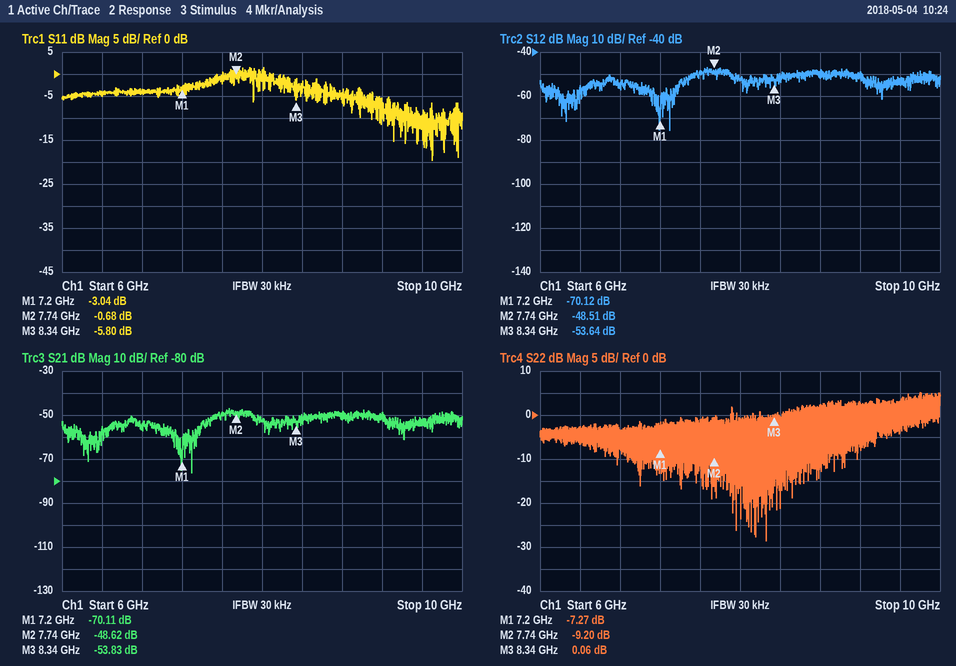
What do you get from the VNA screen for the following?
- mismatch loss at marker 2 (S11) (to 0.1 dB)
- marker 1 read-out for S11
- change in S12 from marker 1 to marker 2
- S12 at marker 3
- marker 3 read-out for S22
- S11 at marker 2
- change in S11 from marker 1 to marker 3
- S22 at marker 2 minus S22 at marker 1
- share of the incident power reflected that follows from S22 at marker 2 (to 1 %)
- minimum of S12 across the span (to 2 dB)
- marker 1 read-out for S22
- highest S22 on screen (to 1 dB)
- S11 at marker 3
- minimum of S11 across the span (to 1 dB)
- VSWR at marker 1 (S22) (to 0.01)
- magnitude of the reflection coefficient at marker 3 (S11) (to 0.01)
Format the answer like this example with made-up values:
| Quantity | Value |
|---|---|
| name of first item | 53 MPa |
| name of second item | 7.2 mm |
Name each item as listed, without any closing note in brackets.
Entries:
| Quantity | Value |
|---|---|
| mismatch loss at marker 2 (S11) | 8.4 dB |
| marker 1 read-out for S11 | -3.04 dB |
| change in S12 from marker 1 to marker 2 | 21.61 dB |
| S12 at marker 3 | -53.64 dB |
| marker 3 read-out for S22 | 0.06 dB |
| S11 at marker 2 | -0.68 dB |
| change in S11 from marker 1 to marker 3 | -2.76 dB |
| S22 at marker 2 minus S22 at marker 1 | -1.93 dB |
| share of the incident power reflected that follows from S22 at marker 2 | 12 % |
| minimum of S12 across the span | -76 dB |
| marker 1 read-out for S22 | -7.27 dB |
| highest S22 on screen | 5 dB |
| S11 at marker 3 | -5.80 dB |
| minimum of S11 across the span | -20 dB |
| VSWR at marker 1 (S22) | 2.53 |
| magnitude of the reflection coefficient at marker 3 (S11) | 0.51 |
